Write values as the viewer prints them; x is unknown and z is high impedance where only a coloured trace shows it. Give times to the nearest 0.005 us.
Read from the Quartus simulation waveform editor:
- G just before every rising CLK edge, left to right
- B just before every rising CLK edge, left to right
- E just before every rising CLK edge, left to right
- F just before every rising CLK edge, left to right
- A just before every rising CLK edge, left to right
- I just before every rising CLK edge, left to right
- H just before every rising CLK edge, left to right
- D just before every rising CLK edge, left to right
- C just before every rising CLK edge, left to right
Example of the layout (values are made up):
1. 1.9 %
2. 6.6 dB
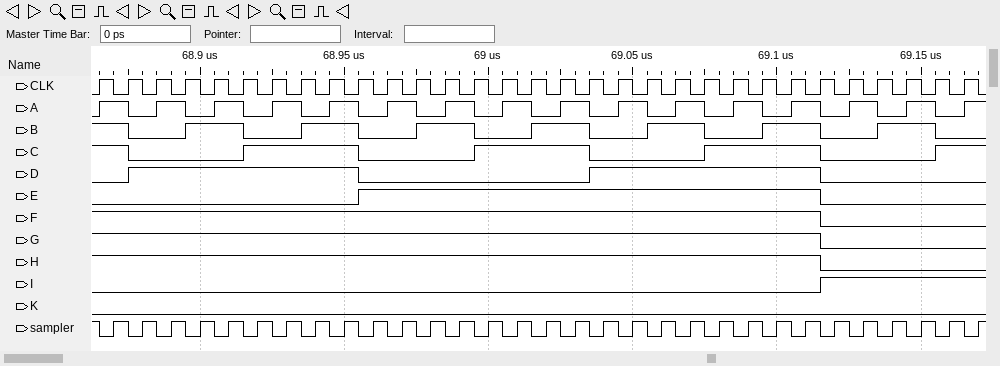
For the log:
1. 1 1 1 1 1 1 1 1 1 1 1 1 1 1 1 1 1 1 1 1 1 1 1 1 1 1 0 0 0 0 0
2. 1 1 0 0 1 1 0 0 1 1 0 0 1 1 0 0 1 1 0 0 1 1 0 0 1 1 0 0 1 1 0
3. 0 0 0 0 0 0 0 0 0 0 1 1 1 1 1 1 1 1 1 1 1 1 1 1 1 1 0 0 0 0 0
4. 1 1 1 1 1 1 1 1 1 1 1 1 1 1 1 1 1 1 1 1 1 1 1 1 1 1 0 0 0 0 0
5. 0 1 0 1 0 1 0 1 0 1 0 1 0 1 0 1 0 1 0 1 0 1 0 1 0 1 0 1 0 1 0
6. 0 0 0 0 0 0 0 0 0 0 0 0 0 0 0 0 0 0 0 0 0 0 0 0 0 0 1 1 1 1 1
7. 1 1 1 1 1 1 1 1 1 1 1 1 1 1 1 1 1 1 1 1 1 1 1 1 1 1 0 0 0 0 0
8. 0 0 1 1 1 1 1 1 1 1 0 0 0 0 0 0 0 0 1 1 1 1 1 1 1 1 0 0 0 0 0
9. 1 1 0 0 0 0 1 1 1 1 0 0 0 0 1 1 1 1 0 0 0 0 1 1 1 1 0 0 0 0 1
